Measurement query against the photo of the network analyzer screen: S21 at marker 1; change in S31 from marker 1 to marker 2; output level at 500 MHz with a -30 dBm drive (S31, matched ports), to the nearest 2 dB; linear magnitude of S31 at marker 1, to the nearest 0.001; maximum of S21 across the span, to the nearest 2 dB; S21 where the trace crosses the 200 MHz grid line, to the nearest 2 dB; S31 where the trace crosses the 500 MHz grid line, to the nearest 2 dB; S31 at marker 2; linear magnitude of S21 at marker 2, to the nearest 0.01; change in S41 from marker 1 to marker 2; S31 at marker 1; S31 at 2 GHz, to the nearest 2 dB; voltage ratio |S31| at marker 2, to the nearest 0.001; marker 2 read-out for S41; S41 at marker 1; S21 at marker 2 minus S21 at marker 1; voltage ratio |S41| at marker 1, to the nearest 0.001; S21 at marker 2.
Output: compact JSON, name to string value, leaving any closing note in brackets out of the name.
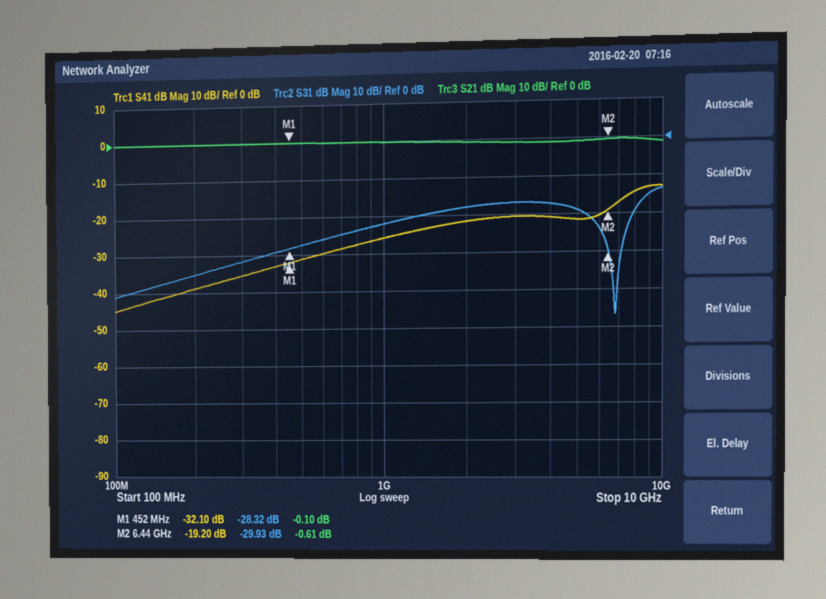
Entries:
{"S21 at marker 1": "-0.10 dB", "change in S31 from marker 1 to marker 2": "-1.61 dB", "output level at 500 MHz with a -30 dBm drive (S31, matched ports), to the nearest 2 dB": "-58 dBm", "linear magnitude of S31 at marker 1, to the nearest 0.001": "0.038", "maximum of S21 across the span, to the nearest 2 dB": "0 dB", "S21 where the trace crosses the 200 MHz grid line, to the nearest 2 dB": "0 dB", "S31 where the trace crosses the 500 MHz grid line, to the nearest 2 dB": "-28 dB", "S31 at marker 2": "-29.93 dB", "linear magnitude of S21 at marker 2, to the nearest 0.01": "0.93", "change in S41 from marker 1 to marker 2": "12.90 dB", "S31 at marker 1": "-28.32 dB", "S31 at 2 GHz, to the nearest 2 dB": "-18 dB", "voltage ratio |S31| at marker 2, to the nearest 0.001": "0.032", "marker 2 read-out for S41": "-19.20 dB", "S41 at marker 1": "-32.10 dB", "S21 at marker 2 minus S21 at marker 1": "-0.51 dB", "voltage ratio |S41| at marker 1, to the nearest 0.001": "0.025", "S21 at marker 2": "-0.61 dB"}
